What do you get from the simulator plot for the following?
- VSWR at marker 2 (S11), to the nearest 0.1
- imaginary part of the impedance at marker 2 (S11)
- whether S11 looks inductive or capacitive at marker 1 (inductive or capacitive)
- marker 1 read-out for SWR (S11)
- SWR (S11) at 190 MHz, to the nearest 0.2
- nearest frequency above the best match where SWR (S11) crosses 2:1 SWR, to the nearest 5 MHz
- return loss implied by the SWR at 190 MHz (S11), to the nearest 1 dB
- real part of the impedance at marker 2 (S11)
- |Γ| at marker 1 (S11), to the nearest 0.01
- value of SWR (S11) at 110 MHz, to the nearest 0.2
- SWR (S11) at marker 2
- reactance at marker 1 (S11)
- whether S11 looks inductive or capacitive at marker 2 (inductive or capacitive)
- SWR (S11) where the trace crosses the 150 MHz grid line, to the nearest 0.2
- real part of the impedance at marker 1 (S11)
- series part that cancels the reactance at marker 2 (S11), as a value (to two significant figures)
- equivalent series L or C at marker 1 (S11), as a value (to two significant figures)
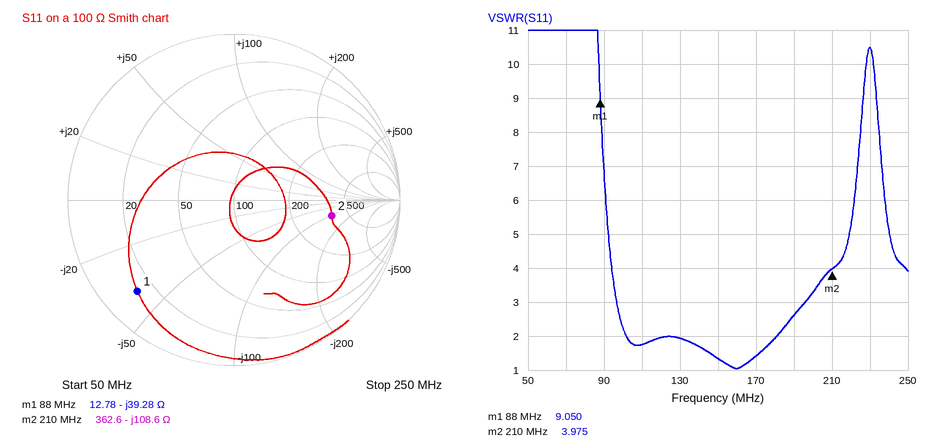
4.0
-108.6 Ω
capacitive
9.050
2.6
180 MHz
7 dB
362.6 Ω
0.80
1.8
3.975
-39.28 Ω
capacitive
1.4
12.78 Ω
82 nH
46 pF
